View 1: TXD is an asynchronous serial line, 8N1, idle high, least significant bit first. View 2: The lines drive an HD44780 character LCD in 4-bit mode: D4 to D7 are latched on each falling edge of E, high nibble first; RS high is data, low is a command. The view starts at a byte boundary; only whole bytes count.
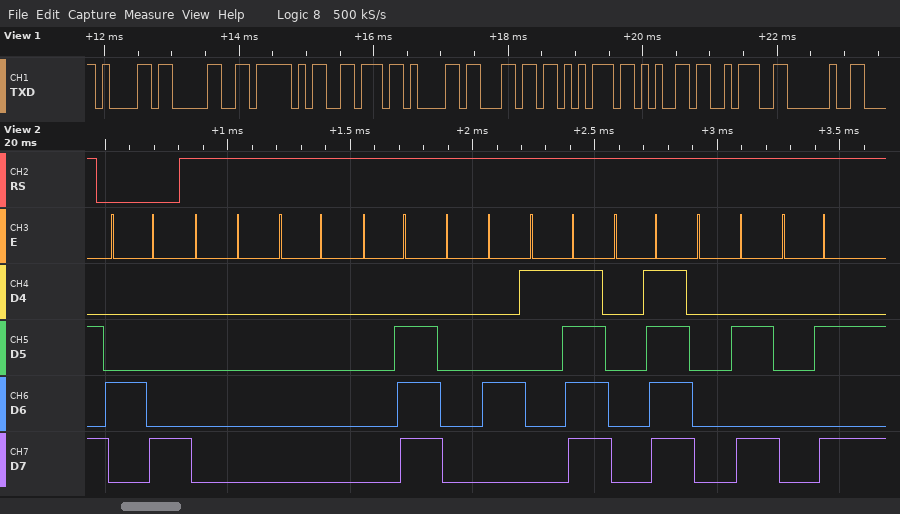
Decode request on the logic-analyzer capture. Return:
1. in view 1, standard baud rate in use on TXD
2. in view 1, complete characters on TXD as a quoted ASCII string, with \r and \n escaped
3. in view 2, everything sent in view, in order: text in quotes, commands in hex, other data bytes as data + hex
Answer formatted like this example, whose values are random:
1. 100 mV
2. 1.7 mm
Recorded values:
1. 9600 baud
2. "a0_value: "
3. 0x48 data 00 00 0E 04 1F 0F 0A 0A
